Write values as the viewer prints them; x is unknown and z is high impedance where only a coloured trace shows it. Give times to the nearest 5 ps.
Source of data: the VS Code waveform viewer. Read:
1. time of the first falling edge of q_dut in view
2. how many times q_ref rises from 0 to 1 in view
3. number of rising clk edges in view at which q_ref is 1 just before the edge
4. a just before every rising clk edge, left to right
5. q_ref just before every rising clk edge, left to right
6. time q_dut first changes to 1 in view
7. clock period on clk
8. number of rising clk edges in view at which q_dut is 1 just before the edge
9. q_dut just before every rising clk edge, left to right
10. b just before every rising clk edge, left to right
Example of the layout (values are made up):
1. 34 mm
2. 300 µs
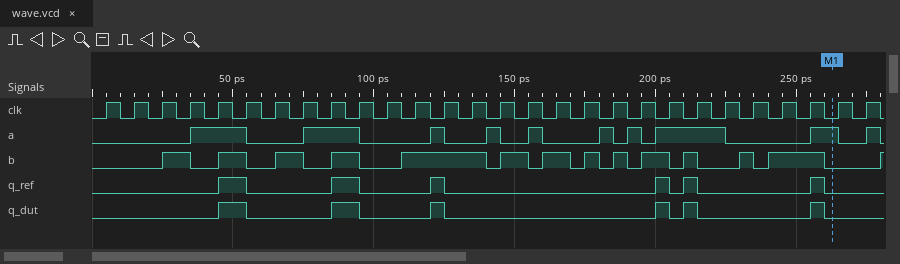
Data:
1. 55 ps
2. 6
3. 5
4. 0 0 0 0 1 1 0 0 1 1 0 0 1 0 1 0 0 0 1 1 1 1 1 0 0 0 1 0
5. 0 0 0 0 0 1 0 0 0 1 0 0 1 0 0 0 0 0 0 0 1 1 0 0 0 0 0 0
6. 45 ps
7. 10 ps
8. 5
9. 0 0 0 0 0 1 0 0 0 1 0 0 1 0 0 0 0 0 0 0 1 1 0 0 0 0 0 0
10. 0 0 0 1 0 1 0 1 0 1 0 1 1 1 0 1 1 0 0 0 1 1 0 1 1 1 0 0
